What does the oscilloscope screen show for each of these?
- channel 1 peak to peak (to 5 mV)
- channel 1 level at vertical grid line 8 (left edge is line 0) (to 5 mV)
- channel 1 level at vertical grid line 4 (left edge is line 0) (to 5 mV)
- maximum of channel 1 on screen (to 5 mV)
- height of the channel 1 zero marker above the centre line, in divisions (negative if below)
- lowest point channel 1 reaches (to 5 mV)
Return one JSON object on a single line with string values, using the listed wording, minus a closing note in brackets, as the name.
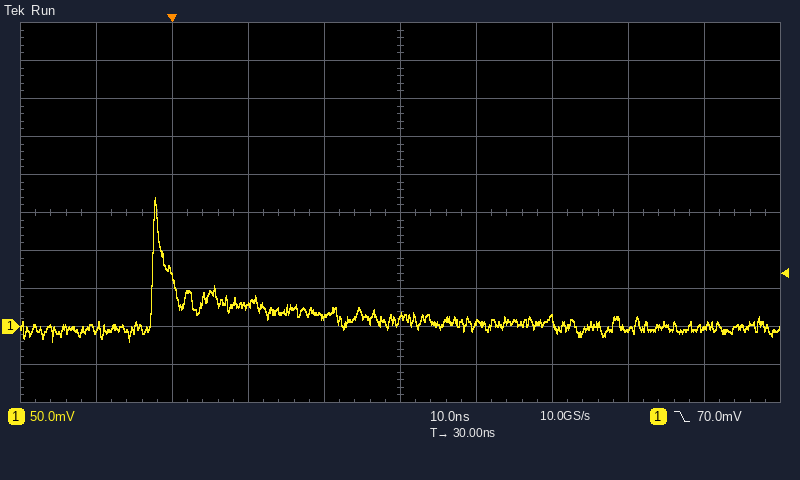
{"channel 1 peak to peak": "190 mV", "channel 1 level at vertical grid line 8 (left edge is line 0)": "-5 mV", "channel 1 level at vertical grid line 4 (left edge is line 0)": "15 mV", "maximum of channel 1 on screen": "170 mV", "height of the channel 1 zero marker above the centre line, in divisions": "-3.0 div", "lowest point channel 1 reaches": "-20 mV"}
